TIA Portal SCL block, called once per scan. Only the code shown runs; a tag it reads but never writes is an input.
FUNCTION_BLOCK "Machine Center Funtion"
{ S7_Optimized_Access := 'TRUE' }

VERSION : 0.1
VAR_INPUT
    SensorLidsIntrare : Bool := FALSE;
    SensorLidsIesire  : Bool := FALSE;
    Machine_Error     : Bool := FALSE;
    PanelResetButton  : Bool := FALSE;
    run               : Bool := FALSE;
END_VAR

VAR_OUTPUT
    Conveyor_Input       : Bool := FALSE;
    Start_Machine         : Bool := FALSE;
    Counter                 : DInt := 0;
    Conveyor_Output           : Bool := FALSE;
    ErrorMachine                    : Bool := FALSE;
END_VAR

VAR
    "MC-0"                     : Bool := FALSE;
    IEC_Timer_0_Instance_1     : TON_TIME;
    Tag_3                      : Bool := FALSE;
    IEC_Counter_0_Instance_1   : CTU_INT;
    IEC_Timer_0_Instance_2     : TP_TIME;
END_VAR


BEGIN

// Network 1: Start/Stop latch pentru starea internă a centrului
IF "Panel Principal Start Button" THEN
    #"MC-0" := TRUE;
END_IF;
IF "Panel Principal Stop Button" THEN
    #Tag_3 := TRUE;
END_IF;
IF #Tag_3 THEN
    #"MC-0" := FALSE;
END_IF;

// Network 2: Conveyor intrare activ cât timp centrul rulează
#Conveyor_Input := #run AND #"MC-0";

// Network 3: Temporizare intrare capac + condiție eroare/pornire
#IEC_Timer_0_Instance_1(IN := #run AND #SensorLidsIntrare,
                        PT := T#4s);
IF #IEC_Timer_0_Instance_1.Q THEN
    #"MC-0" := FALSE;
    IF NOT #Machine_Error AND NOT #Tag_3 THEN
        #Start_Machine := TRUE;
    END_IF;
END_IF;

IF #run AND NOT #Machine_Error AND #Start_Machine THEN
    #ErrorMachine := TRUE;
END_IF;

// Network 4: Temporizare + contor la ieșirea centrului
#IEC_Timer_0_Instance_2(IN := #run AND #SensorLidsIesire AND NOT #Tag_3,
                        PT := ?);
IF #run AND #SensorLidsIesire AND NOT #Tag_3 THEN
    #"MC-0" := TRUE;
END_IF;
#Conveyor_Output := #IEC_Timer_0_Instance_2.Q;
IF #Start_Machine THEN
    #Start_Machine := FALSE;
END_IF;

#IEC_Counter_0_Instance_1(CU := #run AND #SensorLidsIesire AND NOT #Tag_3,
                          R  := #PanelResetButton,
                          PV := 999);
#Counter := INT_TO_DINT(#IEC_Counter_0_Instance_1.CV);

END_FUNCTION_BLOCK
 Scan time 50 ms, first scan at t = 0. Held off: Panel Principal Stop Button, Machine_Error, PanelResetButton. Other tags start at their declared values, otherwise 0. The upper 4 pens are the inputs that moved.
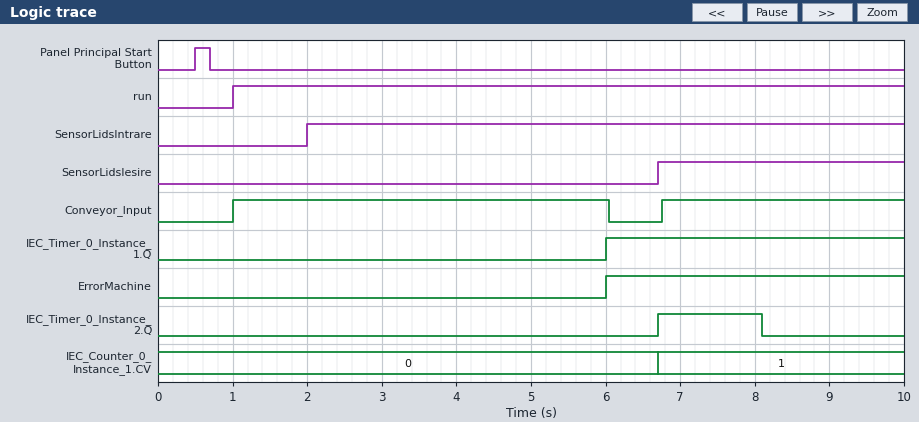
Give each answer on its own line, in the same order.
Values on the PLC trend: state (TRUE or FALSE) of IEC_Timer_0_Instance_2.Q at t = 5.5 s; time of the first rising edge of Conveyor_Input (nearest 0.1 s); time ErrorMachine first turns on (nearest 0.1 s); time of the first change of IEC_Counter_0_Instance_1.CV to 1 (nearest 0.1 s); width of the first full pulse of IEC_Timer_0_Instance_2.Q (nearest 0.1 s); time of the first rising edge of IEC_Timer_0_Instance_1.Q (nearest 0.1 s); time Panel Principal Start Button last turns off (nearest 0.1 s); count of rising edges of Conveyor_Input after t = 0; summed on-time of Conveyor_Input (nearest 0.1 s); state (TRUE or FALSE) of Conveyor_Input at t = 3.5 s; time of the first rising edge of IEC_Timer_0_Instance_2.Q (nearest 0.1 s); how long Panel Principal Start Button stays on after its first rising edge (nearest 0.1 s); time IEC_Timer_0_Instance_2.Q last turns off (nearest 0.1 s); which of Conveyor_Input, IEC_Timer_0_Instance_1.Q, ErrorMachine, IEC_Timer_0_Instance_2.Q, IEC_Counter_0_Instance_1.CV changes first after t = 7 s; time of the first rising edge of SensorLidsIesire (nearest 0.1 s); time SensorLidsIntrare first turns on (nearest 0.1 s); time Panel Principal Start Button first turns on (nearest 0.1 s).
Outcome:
FALSE
1.0 s
6.0 s
6.7 s
1.4 s
6.0 s
0.7 s
2
8.3 s
TRUE
6.7 s
0.2 s
8.1 s
IEC_Timer_0_Instance_2.Q
6.7 s
2.0 s
0.5 s
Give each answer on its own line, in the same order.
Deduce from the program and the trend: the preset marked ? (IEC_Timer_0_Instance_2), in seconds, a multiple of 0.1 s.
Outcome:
1.4 s
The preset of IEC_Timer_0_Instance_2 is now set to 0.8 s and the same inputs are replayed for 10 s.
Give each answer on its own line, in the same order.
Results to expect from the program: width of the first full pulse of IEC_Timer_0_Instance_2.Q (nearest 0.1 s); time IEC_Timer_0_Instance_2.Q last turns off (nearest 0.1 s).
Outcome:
0.8 s
7.5 s
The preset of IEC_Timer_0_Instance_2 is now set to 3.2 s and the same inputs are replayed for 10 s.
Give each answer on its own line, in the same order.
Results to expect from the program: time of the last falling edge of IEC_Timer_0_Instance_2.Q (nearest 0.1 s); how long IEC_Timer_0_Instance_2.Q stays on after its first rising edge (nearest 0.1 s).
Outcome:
9.9 s
3.2 s
